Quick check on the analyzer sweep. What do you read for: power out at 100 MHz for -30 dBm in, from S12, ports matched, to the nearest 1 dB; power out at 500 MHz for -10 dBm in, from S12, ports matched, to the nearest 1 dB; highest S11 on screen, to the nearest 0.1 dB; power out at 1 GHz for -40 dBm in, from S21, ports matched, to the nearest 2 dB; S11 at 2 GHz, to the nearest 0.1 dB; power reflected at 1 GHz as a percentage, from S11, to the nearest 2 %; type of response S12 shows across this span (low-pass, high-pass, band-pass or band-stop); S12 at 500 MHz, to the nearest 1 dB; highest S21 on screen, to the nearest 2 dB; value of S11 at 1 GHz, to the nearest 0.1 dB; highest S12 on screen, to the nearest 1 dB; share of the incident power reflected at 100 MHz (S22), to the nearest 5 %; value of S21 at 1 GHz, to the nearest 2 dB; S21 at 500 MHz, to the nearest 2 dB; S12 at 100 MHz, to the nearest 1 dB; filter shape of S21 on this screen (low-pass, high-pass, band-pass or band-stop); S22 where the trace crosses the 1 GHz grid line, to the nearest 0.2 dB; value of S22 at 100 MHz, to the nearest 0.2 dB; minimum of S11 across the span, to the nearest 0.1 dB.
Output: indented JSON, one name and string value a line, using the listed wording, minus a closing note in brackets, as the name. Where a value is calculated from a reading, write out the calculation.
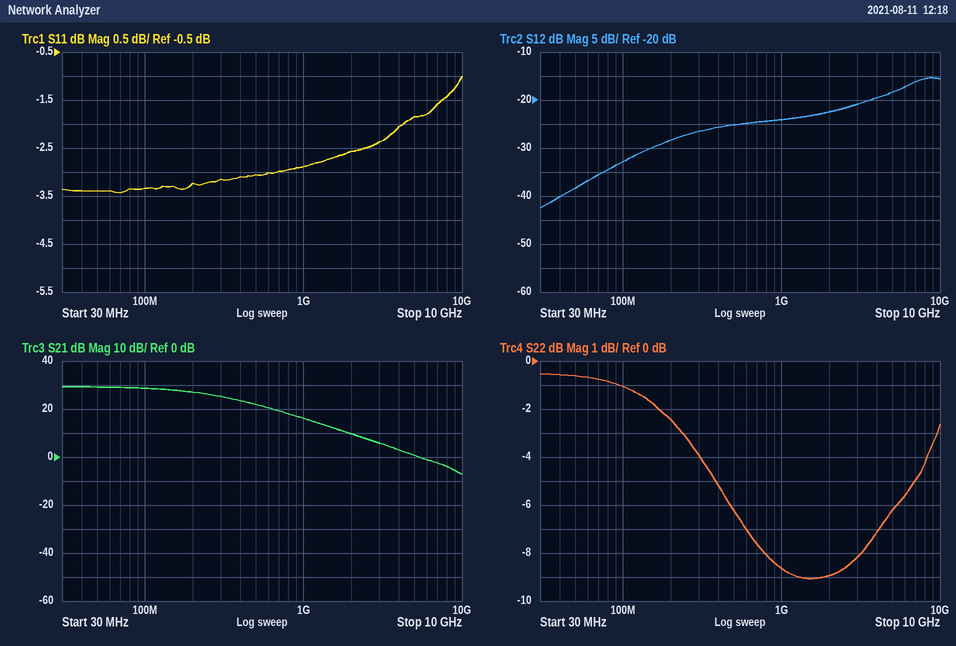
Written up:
{
  "power out at 100 MHz for -30 dBm in, from S12, ports matched, to the nearest 1 dB": "-30 dBm + (-33 dB) = -63 dBm",
  "power out at 500 MHz for -10 dBm in, from S12, ports matched, to the nearest 1 dB": "-10 dBm + (-25 dB) = -35 dBm",
  "highest S11 on screen, to the nearest 0.1 dB": "-1.0 dB",
  "power out at 1 GHz for -40 dBm in, from S21, ports matched, to the nearest 2 dB": "-40 dBm + (16 dB) = -24 dBm",
  "S11 at 2 GHz, to the nearest 0.1 dB": "-2.6 dB",
  "power reflected at 1 GHz as a percentage, from S11, to the nearest 2 %": "10^(-2.9/10) ≈ 51.3 %, so 52 % to the nearest 2 %",
  "type of response S12 shows across this span": "high-pass",
  "S12 at 500 MHz, to the nearest 1 dB": "-25 dB",
  "highest S21 on screen, to the nearest 2 dB": "30 dB",
  "value of S11 at 1 GHz, to the nearest 0.1 dB": "-2.9 dB",
  "highest S12 on screen, to the nearest 1 dB": "-15 dB",
  "share of the incident power reflected at 100 MHz (S22), to the nearest 5 %": "10^(-1/10) ≈ 79.4 %, so 80 % to the nearest 5 %",
  "value of S21 at 1 GHz, to the nearest 2 dB": "16 dB",
  "S21 at 500 MHz, to the nearest 2 dB": "22 dB",
  "S12 at 100 MHz, to the nearest 1 dB": "-33 dB",
  "filter shape of S21 on this screen": "low-pass",
  "S22 where the trace crosses the 1 GHz grid line, to the nearest 0.2 dB": "-8.6 dB",
  "value of S22 at 100 MHz, to the nearest 0.2 dB": "-1.0 dB",
  "minimum of S11 across the span, to the nearest 0.1 dB": "-3.4 dB"
}
